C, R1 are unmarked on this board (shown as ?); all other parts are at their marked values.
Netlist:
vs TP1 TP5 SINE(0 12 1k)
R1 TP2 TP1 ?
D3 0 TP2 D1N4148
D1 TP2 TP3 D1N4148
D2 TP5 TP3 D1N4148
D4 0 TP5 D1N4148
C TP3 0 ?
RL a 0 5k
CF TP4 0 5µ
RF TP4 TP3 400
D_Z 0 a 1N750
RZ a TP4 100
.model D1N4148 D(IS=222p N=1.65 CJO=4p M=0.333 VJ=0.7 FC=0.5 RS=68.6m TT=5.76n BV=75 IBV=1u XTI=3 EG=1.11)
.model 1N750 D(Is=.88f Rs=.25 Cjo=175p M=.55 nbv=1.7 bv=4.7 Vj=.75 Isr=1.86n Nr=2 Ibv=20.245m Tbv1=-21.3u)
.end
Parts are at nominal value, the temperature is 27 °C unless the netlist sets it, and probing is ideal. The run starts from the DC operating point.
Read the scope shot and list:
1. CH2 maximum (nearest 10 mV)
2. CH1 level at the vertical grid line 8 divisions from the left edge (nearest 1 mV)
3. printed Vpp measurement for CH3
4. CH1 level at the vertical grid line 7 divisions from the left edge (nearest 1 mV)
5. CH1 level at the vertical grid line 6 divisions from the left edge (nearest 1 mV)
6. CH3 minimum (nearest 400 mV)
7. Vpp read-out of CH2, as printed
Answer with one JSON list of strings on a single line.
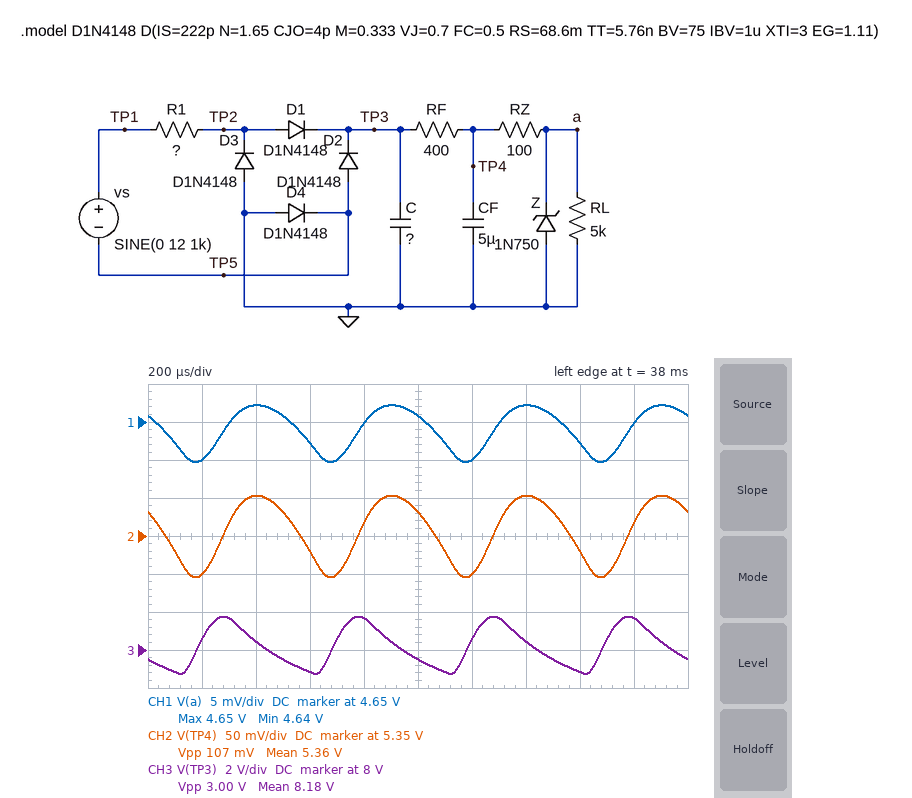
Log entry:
["5.40 V", "4.647 V", "3.00 V", "4.652 V", "4.645 V", "6.8 V", "107 mV"]
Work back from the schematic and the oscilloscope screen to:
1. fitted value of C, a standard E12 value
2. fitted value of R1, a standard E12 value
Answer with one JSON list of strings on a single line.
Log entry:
["680 nF", "47 Ω"]
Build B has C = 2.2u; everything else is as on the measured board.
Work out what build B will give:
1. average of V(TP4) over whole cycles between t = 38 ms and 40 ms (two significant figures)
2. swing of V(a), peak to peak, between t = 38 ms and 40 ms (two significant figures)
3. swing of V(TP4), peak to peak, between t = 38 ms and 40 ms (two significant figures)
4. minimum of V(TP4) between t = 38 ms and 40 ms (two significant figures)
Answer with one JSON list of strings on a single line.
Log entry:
["5.5 V", "2.5 mV", "41 mV", "5.4 V"]
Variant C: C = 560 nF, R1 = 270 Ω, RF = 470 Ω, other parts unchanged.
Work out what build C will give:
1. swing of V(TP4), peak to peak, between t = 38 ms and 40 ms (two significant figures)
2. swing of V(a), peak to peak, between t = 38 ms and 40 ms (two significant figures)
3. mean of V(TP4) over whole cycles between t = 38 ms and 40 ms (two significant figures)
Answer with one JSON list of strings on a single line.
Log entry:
["56 mV", "7.0 mV", "5.0 V"]
